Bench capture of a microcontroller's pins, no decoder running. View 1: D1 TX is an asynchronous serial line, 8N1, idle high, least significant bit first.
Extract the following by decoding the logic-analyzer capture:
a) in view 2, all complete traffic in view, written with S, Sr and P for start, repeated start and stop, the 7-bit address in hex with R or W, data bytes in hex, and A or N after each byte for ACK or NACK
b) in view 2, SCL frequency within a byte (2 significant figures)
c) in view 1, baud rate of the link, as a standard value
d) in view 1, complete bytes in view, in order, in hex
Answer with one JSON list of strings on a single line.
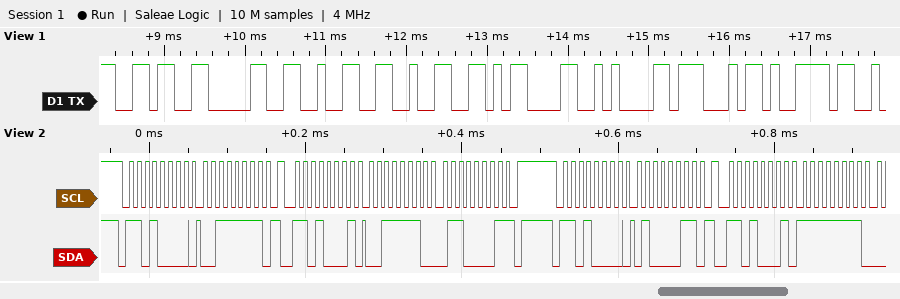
["S 68W A 3F A Sr 68R A 3E A 61 N P S 68W A 43 A Sr 68R A FF A", "100 kHz", "9600 baud", "36 30 32 32 0D 0A 47 79"]
